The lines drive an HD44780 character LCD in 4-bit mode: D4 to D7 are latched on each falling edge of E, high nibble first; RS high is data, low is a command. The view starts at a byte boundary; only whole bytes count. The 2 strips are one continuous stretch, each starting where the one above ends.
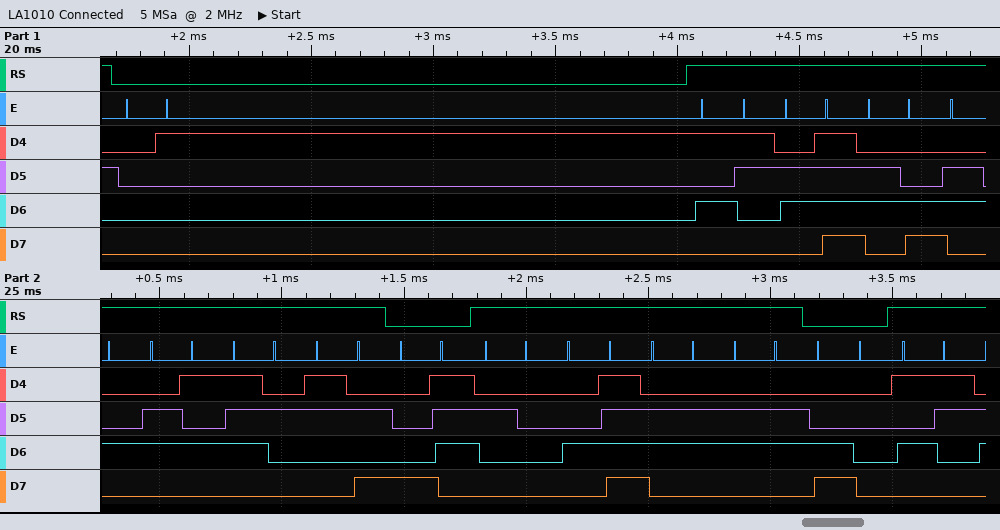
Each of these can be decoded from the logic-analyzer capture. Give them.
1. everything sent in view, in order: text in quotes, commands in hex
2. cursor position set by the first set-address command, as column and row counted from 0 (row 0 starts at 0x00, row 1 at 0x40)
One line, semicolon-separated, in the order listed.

0x01 "Solder:" 0x87 " Off" 0xC0 "S"; column 7, row 0
